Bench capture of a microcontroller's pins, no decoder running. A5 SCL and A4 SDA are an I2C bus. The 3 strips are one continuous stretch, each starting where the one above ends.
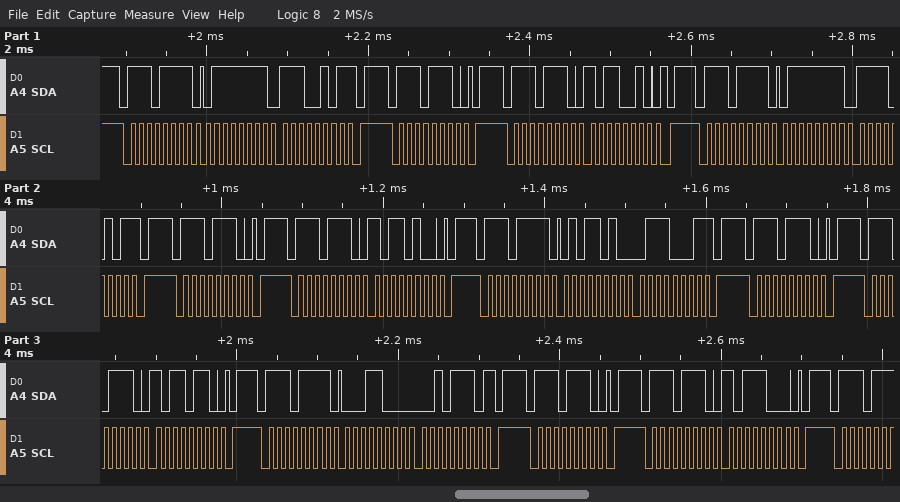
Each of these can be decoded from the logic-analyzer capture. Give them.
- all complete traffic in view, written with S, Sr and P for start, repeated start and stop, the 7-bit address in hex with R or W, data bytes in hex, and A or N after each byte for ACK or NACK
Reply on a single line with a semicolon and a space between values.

S 77R A 7F A E5 N P S 77W A P S 77W A B2 A P S 77R A 7F A F5 N P S 77W A P S 77W A B4 A P S 77R A 5A A 71 N P S 77W A P S 77W A B6 A P S 77R A 18 A 2E N P S 77W A P S 77W A B8 A P
